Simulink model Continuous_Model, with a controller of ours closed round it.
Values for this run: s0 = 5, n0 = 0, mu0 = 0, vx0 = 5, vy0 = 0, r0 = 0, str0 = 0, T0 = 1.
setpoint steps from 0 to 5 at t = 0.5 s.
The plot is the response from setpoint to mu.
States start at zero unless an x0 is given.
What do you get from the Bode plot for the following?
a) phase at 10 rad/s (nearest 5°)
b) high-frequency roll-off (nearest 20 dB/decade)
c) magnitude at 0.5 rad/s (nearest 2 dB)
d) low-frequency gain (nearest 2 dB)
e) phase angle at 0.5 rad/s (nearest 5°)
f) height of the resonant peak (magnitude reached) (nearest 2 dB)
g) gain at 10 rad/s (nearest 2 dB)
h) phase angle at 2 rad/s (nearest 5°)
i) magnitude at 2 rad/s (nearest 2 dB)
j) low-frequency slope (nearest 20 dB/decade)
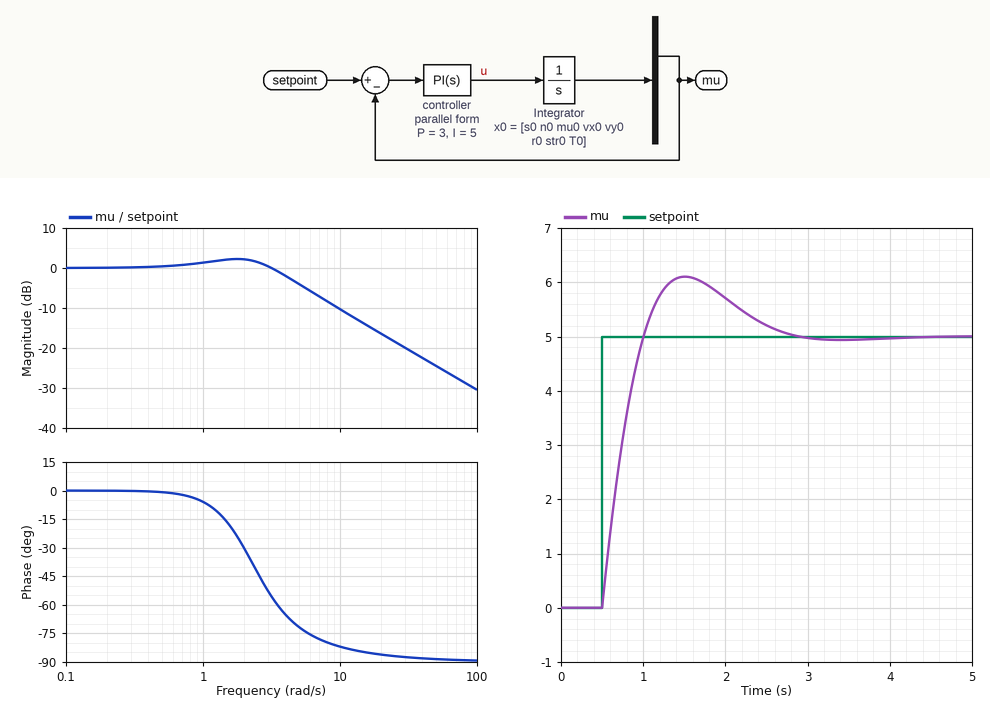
-80°
-20 dB/decade
0 dB
0 dB
0°
2 dB
-10 dB
-30°
2 dB
0 dB/decade
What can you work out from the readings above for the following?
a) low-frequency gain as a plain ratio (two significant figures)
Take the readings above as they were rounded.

1.0
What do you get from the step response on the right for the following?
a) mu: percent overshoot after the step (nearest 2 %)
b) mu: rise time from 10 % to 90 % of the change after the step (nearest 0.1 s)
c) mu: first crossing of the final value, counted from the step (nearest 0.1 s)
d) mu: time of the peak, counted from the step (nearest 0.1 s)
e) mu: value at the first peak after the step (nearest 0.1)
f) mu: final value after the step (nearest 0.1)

22 %
0.4 s
0.5 s
1.0 s
6.1
5.0
